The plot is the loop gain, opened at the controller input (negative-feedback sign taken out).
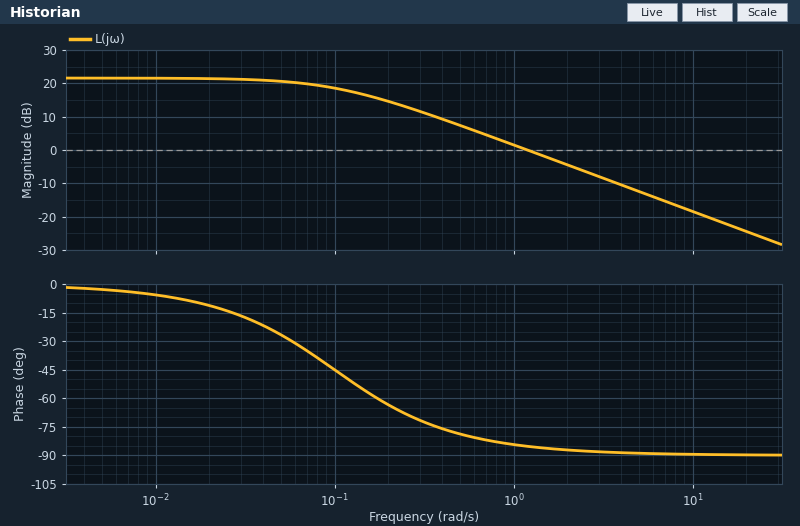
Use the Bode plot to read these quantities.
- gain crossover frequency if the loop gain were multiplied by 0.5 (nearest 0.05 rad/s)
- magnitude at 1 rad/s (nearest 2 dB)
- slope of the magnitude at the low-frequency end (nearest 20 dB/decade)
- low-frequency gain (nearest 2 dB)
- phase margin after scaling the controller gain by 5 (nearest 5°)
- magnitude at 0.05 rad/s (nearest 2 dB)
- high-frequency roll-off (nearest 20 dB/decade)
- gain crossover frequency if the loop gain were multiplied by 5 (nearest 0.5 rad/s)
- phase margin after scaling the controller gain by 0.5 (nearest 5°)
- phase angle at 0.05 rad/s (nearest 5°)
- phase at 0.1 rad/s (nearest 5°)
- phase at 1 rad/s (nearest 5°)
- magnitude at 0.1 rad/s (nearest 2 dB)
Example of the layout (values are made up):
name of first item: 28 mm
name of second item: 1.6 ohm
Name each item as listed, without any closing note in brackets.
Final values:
gain crossover frequency if the loop gain were multiplied by 0.5: 0.60 rad/s
magnitude at 1 rad/s: 2 dB
slope of the magnitude at the low-frequency end: 0 dB/decade
low-frequency gain: 22 dB
phase margin after scaling the controller gain by 5: 90°
magnitude at 0.05 rad/s: 20 dB
high-frequency roll-off: -20 dB/decade
gain crossover frequency if the loop gain were multiplied by 5: 6.0 rad/s
phase margin after scaling the controller gain by 0.5: 100°
phase angle at 0.05 rad/s: -25°
phase at 0.1 rad/s: -45°
phase at 1 rad/s: -85°
magnitude at 0.1 rad/s: 18 dB
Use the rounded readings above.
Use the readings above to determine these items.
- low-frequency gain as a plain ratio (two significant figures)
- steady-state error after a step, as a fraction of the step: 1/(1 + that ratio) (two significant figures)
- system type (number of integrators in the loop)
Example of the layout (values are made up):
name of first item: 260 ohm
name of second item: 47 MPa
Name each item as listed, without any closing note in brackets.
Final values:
low-frequency gain as a plain ratio: 13
steady-state error after a step, as a fraction of the step: 1/(1 + that ratio): 0.071
system type: 0
